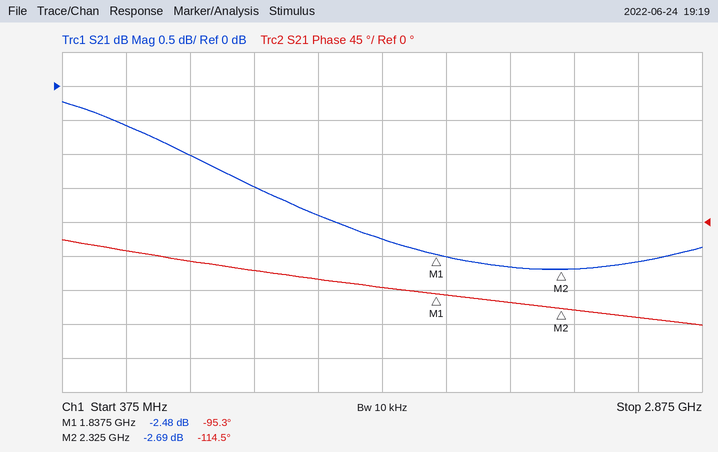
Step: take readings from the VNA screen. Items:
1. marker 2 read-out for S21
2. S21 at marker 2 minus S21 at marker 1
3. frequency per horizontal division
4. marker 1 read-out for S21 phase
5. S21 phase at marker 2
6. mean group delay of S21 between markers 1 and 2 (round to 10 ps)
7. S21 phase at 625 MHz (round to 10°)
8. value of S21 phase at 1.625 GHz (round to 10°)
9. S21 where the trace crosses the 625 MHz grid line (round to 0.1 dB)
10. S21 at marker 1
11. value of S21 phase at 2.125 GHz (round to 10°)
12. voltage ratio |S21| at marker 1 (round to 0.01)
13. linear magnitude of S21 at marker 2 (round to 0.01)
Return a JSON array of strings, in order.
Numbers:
["-2.69 dB", "-0.21 dB", "250 MHz", "-95.3°", "-114.5°", "110 ps", "-40°", "-90°", "-0.6 dB", "-2.48 dB", "-110°", "0.75", "0.73"]
